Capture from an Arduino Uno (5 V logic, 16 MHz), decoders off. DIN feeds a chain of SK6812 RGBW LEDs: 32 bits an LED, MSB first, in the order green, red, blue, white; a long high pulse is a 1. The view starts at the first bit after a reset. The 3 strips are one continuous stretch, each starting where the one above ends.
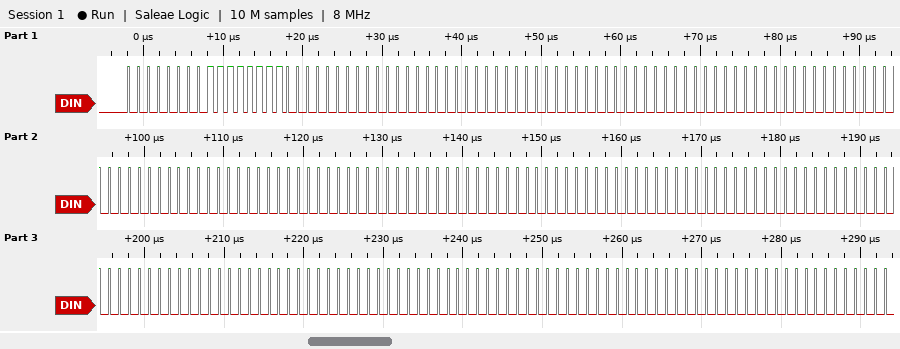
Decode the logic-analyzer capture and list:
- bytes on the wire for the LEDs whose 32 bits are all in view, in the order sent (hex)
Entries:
00 FF 00 00 00 00 00 00 00 00 00 00 00 00 00 00 00 00 00 00 00 00 00 00 00 00 00 00
